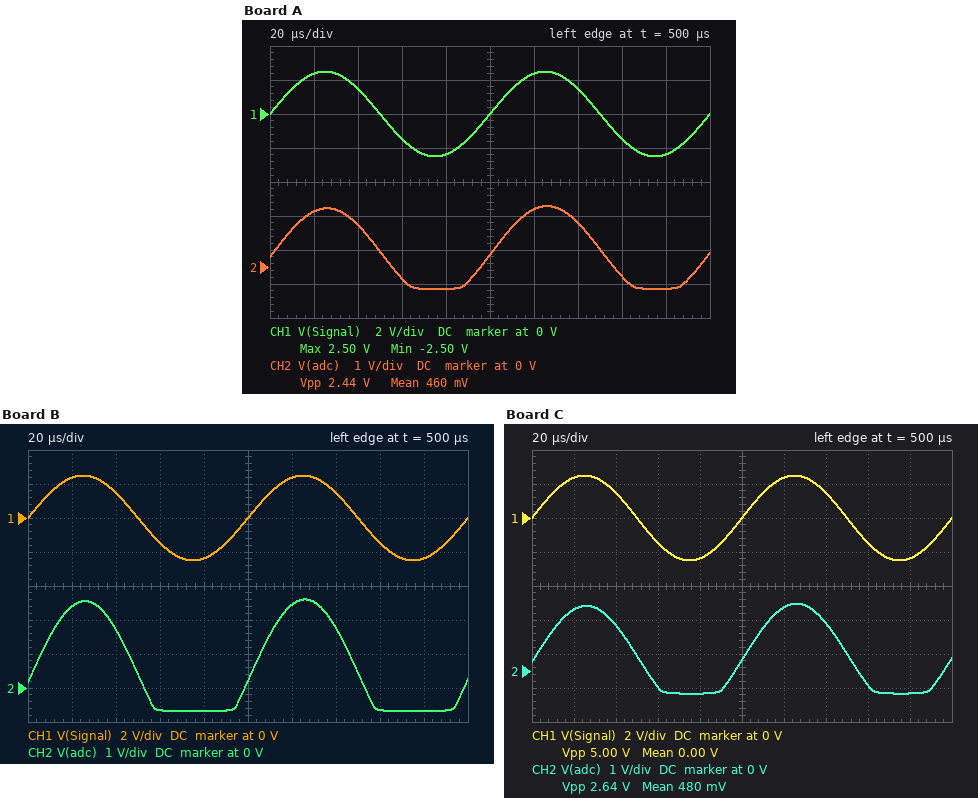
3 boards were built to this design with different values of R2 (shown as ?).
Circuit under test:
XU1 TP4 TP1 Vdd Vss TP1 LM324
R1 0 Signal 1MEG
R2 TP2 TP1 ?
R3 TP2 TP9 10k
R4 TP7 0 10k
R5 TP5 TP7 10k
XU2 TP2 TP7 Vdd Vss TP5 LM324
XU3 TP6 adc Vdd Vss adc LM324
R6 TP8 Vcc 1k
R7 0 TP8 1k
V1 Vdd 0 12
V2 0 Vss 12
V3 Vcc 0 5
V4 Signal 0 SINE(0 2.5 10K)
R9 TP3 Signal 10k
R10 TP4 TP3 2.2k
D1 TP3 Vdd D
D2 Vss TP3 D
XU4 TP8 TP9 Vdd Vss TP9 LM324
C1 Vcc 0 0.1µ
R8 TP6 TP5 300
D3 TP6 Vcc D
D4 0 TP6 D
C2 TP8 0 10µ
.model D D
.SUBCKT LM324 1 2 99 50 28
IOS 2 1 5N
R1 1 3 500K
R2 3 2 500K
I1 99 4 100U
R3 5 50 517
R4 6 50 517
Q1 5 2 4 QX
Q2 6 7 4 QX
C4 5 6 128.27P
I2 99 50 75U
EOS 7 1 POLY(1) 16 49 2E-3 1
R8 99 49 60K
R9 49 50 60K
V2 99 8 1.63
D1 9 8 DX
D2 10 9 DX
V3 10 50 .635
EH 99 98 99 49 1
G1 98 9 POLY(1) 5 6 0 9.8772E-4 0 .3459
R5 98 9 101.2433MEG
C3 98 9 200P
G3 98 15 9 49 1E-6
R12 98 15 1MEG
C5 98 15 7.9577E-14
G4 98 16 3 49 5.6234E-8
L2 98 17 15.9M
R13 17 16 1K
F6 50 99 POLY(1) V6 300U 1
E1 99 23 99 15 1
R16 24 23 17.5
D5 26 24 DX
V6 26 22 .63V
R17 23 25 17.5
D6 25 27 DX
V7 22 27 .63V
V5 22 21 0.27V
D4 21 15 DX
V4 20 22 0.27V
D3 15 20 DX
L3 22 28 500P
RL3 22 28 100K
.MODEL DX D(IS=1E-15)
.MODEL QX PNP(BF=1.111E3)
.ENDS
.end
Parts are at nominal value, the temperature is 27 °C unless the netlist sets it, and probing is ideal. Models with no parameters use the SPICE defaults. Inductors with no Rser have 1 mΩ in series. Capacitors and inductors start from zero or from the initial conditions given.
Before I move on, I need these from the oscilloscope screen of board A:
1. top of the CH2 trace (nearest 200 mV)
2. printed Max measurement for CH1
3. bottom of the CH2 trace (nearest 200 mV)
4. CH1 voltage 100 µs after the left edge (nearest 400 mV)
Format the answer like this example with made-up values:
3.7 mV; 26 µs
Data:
1.8 V; 2.50 V; -600 mV; 0 V
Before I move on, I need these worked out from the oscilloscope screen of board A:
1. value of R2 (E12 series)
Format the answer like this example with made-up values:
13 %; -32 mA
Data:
27 kΩ
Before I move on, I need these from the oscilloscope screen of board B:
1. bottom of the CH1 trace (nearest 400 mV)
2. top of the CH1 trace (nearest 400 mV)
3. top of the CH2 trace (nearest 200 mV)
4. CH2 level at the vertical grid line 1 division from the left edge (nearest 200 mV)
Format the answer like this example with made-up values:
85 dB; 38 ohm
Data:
-2.4 V; 2.4 V; 2.6 V; 2.4 V
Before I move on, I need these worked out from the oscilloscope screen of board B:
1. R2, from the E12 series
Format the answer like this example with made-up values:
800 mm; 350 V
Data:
12 kΩ
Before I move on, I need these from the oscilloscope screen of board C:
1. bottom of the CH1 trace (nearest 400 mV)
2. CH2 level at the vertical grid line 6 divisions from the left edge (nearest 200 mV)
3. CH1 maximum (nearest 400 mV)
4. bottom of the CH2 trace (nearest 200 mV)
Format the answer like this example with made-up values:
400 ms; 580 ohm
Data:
-2.4 V; 1.8 V; 2.4 V; -600 mV
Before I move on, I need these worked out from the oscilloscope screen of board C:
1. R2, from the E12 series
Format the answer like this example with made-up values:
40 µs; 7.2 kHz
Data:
22 kΩ
